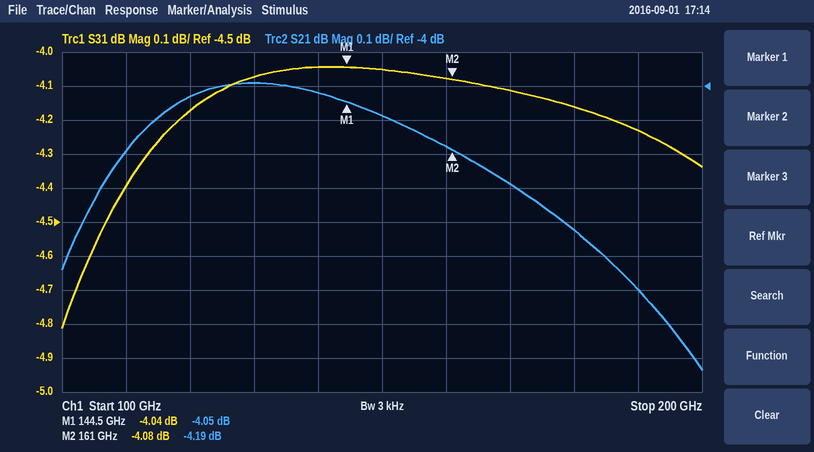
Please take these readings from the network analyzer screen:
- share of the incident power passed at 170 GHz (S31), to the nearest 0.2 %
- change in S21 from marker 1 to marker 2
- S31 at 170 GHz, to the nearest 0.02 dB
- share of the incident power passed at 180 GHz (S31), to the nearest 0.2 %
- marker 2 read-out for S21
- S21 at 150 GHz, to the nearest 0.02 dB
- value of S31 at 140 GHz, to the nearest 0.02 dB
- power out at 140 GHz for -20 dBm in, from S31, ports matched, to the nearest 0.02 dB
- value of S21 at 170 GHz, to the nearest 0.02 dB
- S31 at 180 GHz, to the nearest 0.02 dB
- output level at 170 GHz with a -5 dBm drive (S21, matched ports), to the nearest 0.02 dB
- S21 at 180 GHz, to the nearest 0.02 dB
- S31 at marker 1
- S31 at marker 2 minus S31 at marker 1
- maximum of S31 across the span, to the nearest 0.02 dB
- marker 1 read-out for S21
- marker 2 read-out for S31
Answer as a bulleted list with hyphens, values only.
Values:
- 38.8 %
- -0.14 dB
- -4.12 dB
- 38.4 %
- -4.19 dB
- -4.08 dB
- -4.04 dB
- -24.04 dBm
- -4.28 dB
- -4.16 dB
- -9.28 dBm
- -4.42 dB
- -4.04 dB
- -0.04 dB
- -4.04 dB
- -4.05 dB
- -4.08 dB
